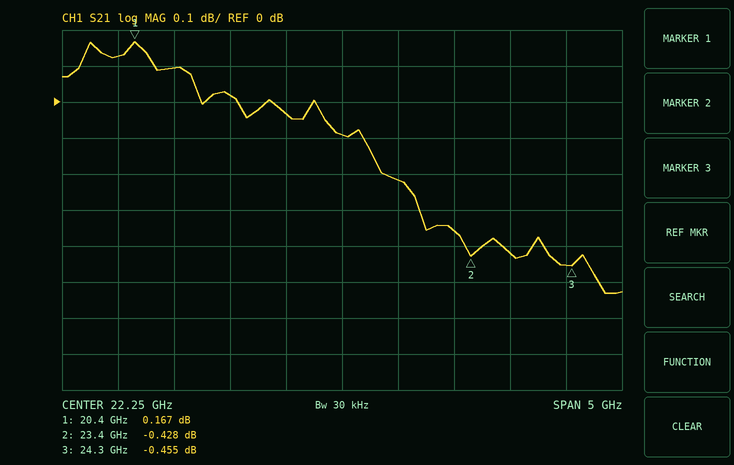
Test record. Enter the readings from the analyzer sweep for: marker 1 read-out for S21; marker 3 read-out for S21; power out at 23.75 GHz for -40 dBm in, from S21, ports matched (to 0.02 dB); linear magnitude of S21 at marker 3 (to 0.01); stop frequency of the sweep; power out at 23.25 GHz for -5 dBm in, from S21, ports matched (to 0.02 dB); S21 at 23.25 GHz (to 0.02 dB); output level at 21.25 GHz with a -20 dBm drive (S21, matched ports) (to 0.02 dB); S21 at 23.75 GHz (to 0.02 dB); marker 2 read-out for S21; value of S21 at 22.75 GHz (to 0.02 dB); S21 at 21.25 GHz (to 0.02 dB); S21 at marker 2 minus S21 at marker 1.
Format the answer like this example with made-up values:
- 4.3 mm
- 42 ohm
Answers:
- 0.167 dB
- -0.455 dB
- -40.42 dBm
- 0.95
- 24.75 GHz
- -5.36 dBm
- -0.36 dB
- -19.98 dBm
- -0.42 dB
- -0.428 dB
- -0.22 dB
- 0.02 dB
- -0.595 dB
